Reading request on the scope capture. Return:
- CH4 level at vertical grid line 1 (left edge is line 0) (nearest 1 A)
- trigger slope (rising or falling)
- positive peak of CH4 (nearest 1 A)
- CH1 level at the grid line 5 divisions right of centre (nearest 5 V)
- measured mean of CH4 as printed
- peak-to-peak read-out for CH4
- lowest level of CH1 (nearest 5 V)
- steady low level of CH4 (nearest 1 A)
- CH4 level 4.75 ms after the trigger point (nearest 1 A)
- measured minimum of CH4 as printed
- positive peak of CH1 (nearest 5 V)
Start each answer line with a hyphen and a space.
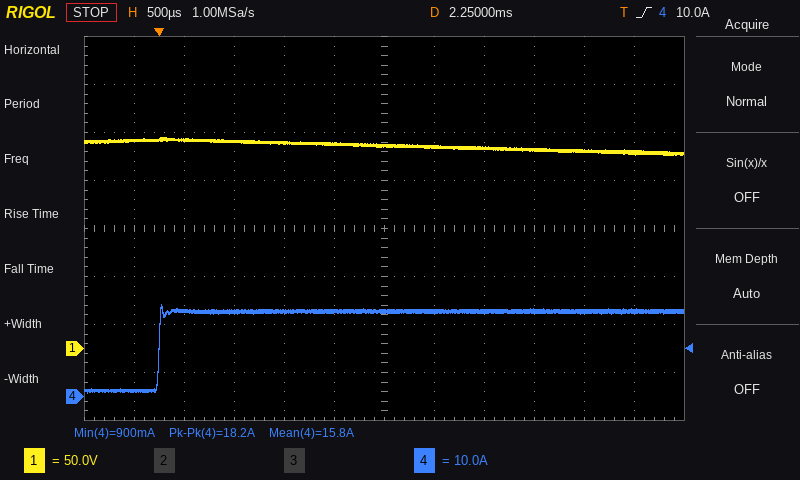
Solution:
- 1 A
- rising
- 19 A
- 205 V
- 15.8 A
- 18.2 A
- 200 V
- 1 A
- 18 A
- 900 mA
- 220 V
